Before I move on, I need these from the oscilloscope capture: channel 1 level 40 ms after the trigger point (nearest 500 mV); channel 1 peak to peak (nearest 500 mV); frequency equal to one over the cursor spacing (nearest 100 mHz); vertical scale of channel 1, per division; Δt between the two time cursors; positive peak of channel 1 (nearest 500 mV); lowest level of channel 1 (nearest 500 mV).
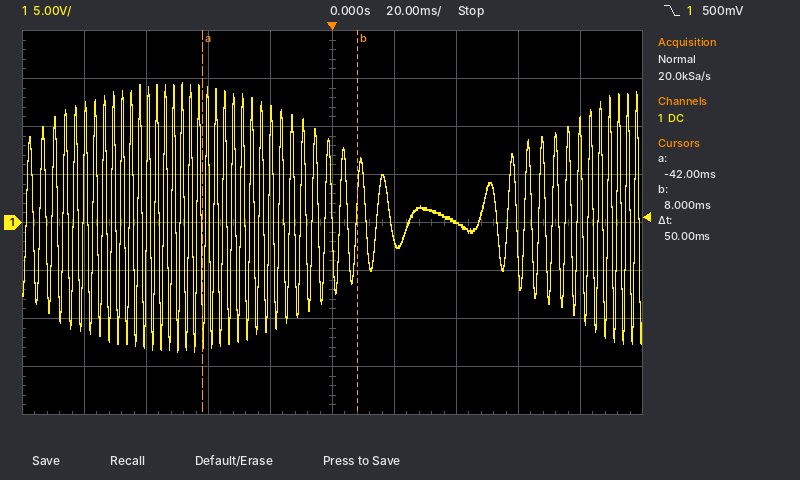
0.0 V
28.0 V
20.0 Hz
5 V
50 ms
14.5 V
-13.5 V
